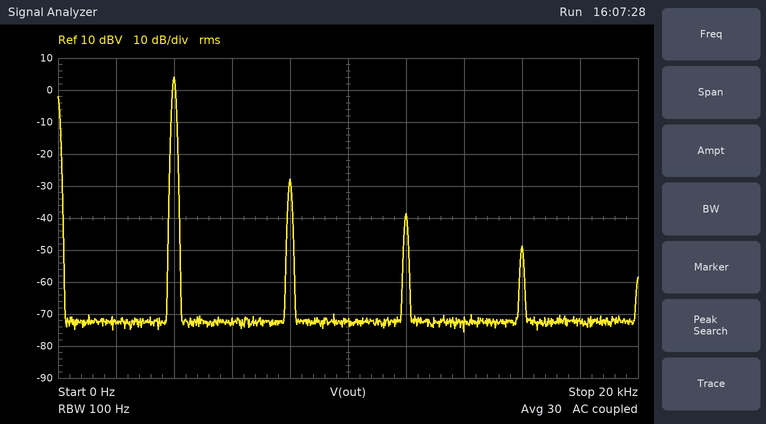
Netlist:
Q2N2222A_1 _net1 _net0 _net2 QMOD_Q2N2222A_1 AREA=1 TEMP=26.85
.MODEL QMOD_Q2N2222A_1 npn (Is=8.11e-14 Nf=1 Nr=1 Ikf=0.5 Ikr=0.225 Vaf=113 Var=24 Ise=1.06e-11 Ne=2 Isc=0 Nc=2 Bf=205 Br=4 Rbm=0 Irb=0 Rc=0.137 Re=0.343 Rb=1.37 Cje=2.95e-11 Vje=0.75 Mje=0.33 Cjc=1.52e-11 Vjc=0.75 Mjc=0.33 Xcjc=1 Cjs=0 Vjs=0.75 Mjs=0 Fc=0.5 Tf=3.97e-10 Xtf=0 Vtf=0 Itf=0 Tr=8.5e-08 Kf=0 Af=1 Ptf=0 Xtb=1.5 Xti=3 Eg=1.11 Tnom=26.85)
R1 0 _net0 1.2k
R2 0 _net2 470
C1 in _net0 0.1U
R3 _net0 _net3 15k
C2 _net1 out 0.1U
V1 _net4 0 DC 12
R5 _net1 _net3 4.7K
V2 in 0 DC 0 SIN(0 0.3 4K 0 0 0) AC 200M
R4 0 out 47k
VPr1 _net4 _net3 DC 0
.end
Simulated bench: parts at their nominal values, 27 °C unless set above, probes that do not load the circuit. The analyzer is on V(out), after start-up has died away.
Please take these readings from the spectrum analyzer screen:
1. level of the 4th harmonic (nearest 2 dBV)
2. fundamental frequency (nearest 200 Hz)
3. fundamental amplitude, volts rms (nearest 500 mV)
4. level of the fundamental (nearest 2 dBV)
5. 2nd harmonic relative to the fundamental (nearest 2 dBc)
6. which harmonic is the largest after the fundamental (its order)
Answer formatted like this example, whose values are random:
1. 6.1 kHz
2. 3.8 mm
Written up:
1. -48 dBV
2. 4.0 kHz
3. 1.5 V
4. 4 dBV
5. -32 dBc
6. 2
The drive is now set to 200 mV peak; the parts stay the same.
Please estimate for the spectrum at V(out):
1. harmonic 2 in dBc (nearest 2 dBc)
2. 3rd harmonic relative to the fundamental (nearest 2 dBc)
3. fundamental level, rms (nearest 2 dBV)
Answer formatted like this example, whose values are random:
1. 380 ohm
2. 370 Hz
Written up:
1. -38 dBc
2. -52 dBc
3. 0 dBV
